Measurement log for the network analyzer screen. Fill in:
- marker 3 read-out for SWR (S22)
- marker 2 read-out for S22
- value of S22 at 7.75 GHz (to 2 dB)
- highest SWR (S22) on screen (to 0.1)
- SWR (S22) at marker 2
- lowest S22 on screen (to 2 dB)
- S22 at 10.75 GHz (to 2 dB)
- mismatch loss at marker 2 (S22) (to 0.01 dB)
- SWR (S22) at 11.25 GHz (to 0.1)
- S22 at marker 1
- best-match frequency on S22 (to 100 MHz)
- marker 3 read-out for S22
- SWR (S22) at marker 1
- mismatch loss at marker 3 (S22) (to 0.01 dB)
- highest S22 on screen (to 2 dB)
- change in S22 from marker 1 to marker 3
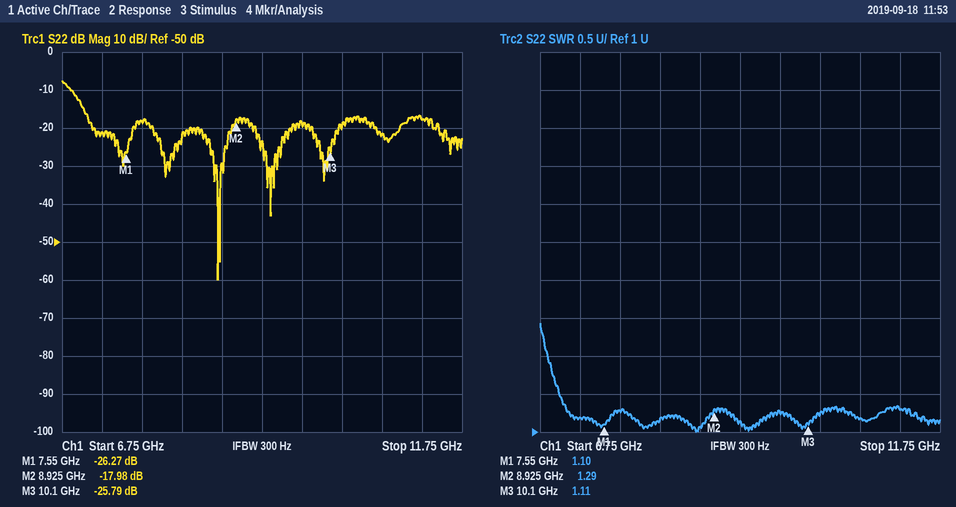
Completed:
1.11
-17.98 dB
-18 dB
2.4
1.29
-60 dB
-22 dB
0.07 dB
1.3
-26.27 dB
8.7 GHz
-25.79 dB
1.10
0.01 dB
-8 dB
0.48 dB
